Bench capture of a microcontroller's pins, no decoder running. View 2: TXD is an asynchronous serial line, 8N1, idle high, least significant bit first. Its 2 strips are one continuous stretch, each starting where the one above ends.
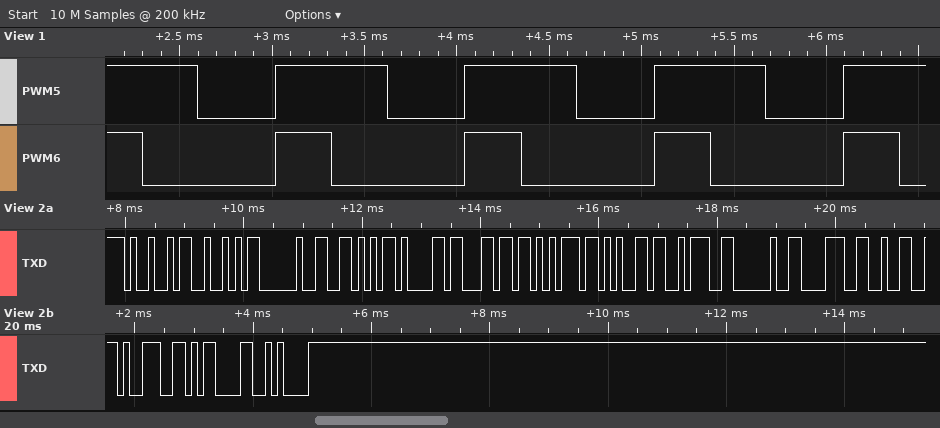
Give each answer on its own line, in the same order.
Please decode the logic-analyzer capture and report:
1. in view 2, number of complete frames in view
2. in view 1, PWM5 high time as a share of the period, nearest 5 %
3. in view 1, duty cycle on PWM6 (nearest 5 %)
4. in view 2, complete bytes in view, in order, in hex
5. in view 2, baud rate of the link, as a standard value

15
60 %
30 %
0x49 0x52 0x20 0x56 0x61 0x6C 0x75 0x65 0x3A 0x20 0x38 0x32 0x39 0x0D 0x0A
9600 baud
